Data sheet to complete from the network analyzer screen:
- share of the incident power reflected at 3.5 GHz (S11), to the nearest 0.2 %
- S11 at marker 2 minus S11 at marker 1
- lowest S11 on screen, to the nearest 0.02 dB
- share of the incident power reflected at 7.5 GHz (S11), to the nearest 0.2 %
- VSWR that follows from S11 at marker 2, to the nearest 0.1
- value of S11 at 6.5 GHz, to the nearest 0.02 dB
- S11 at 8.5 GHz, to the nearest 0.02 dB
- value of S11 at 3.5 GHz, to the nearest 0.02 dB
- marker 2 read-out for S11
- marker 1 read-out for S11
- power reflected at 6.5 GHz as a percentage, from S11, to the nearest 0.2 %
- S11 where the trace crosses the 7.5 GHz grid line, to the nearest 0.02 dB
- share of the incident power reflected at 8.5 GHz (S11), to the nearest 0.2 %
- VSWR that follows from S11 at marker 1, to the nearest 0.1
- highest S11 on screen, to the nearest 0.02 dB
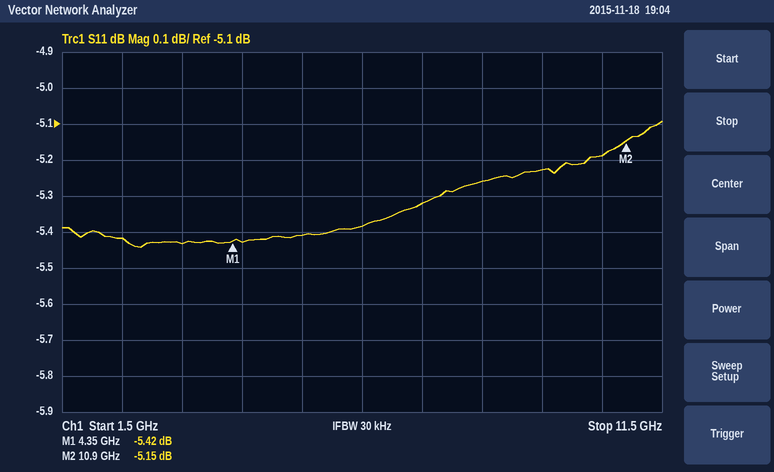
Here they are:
28.6 %
0.27 dB
-5.44 dB
29.4 %
3.5
-5.38 dB
-5.26 dB
-5.44 dB
-5.15 dB
-5.42 dB
29.0 %
-5.32 dB
29.8 %
3.3
-5.10 dB
